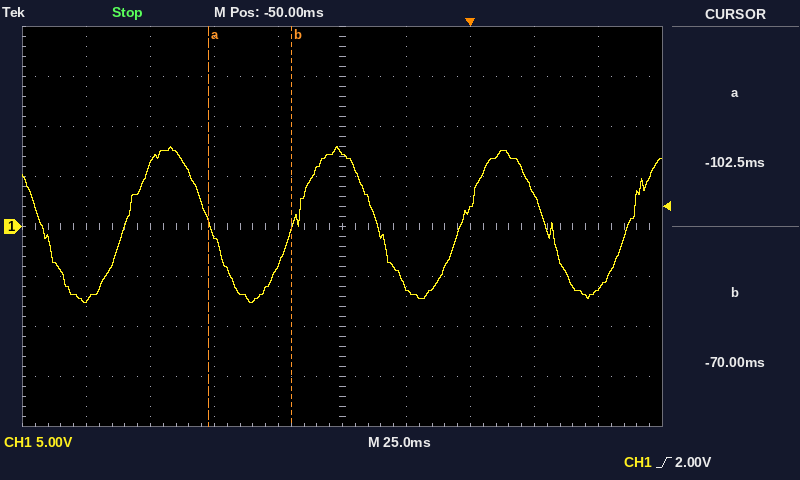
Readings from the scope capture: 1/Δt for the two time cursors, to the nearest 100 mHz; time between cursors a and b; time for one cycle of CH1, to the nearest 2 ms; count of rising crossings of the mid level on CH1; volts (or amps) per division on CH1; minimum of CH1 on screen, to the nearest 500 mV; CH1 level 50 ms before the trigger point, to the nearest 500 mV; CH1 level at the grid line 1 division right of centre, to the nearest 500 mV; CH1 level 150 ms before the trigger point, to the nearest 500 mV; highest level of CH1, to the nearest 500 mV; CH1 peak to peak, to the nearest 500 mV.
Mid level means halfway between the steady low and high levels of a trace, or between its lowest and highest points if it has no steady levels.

30.8 Hz
32.5 ms
66 ms
4
5 V
-7.5 V
7.5 V
-6.0 V
-7.5 V
8.0 V
15.5 V
